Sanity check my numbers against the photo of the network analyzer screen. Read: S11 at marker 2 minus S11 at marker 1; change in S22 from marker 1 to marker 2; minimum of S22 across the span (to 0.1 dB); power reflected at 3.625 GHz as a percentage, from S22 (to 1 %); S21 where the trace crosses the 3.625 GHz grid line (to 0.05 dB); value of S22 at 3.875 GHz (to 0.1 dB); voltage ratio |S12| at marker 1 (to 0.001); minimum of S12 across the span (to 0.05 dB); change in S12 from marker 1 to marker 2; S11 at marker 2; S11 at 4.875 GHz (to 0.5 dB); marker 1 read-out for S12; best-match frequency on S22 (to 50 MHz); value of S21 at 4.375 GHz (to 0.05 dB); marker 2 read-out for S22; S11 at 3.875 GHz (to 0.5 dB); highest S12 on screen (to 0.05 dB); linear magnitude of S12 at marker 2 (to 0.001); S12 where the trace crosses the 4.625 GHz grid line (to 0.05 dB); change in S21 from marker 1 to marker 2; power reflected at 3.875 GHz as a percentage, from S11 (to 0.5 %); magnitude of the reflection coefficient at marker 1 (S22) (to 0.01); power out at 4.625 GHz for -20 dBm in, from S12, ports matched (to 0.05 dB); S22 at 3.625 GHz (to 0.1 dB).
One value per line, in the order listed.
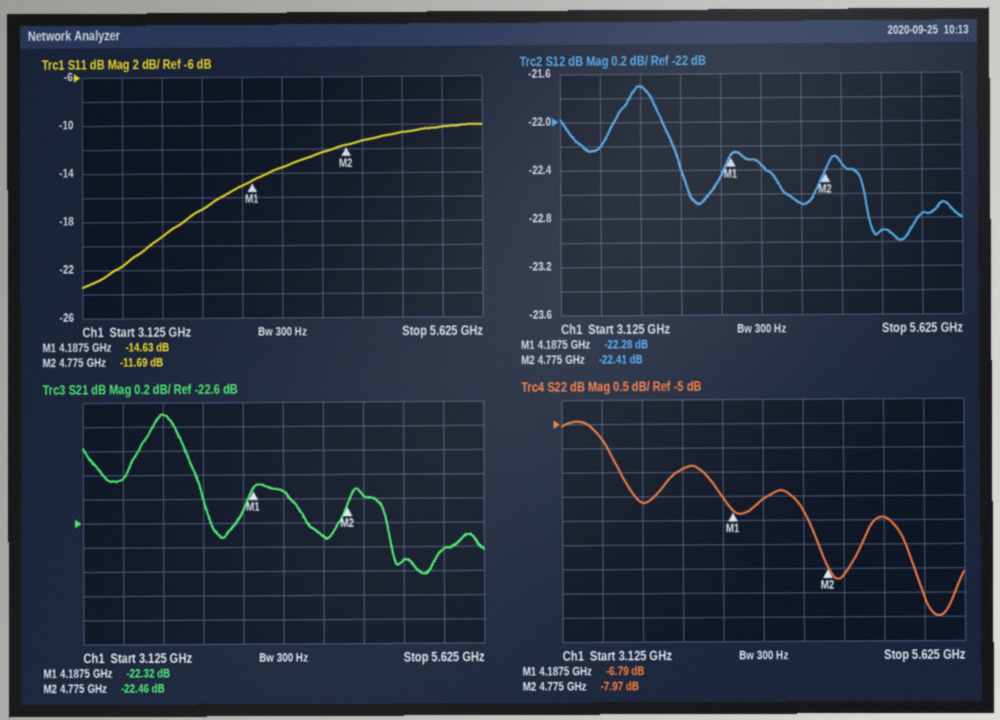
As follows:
2.94 dB
-1.18 dB
-9.0 dB
22 %
-21.70 dB
-5.9 dB
0.077
-23.00 dB
-0.13 dB
-11.69 dB
-11.5 dB
-22.28 dB
5.45 GHz
-22.35 dB
-7.97 dB
-17.0 dB
-21.70 dB
0.076
-22.70 dB
-0.14 dB
2.0 %
0.46
-42.70 dBm
-6.6 dB
